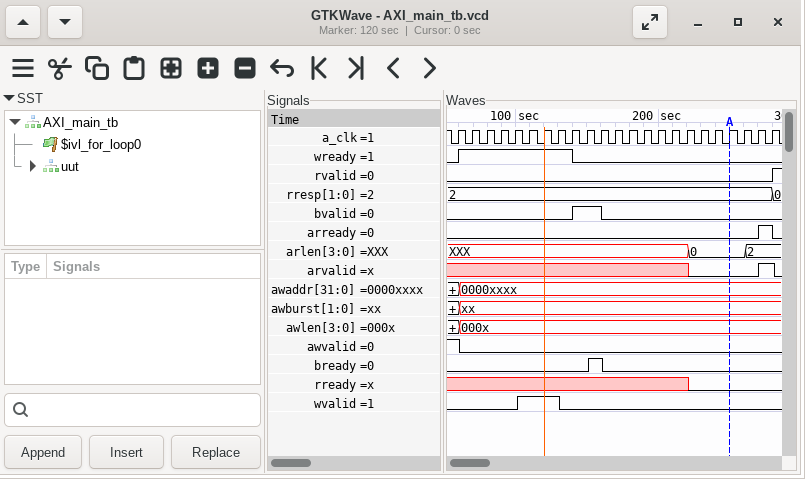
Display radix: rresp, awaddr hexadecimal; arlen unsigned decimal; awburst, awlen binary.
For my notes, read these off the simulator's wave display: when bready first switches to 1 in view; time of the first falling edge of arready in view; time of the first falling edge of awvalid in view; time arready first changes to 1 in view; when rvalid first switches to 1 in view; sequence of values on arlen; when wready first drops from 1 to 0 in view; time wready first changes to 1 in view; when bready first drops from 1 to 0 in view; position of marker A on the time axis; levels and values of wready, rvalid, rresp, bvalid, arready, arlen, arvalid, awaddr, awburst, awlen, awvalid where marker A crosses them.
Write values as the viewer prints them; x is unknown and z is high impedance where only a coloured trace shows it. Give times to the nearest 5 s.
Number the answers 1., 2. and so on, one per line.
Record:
1. 150 s
2. 280 s
3. 60 s
4. 270 s
5. 280 s
6. XXX, 0, 2
7. 140 s
8. 60 s
9. 160 s
10. 250 s
11. wready=0, rvalid=0, rresp=2, bvalid=0, arready=0, arlen=0, arvalid=0, awaddr=0000xxxx, awburst=xx, awlen=000x, awvalid=0
